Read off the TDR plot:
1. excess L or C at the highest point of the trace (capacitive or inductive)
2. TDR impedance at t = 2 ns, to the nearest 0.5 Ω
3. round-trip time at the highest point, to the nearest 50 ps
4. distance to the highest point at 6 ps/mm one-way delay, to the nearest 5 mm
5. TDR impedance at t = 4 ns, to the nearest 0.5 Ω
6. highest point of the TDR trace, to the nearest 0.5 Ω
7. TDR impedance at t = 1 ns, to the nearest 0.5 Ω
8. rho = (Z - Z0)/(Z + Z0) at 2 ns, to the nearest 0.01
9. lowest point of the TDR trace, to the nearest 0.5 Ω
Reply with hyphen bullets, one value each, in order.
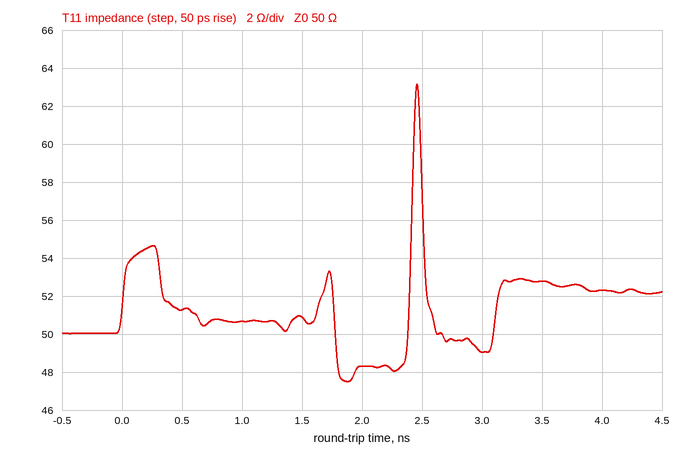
- inductive
- 48.5 Ω
- 2.45 ns
- 205 mm
- 52.5 Ω
- 63.0 Ω
- 50.5 Ω
- -0.02
- 47.5 Ω
